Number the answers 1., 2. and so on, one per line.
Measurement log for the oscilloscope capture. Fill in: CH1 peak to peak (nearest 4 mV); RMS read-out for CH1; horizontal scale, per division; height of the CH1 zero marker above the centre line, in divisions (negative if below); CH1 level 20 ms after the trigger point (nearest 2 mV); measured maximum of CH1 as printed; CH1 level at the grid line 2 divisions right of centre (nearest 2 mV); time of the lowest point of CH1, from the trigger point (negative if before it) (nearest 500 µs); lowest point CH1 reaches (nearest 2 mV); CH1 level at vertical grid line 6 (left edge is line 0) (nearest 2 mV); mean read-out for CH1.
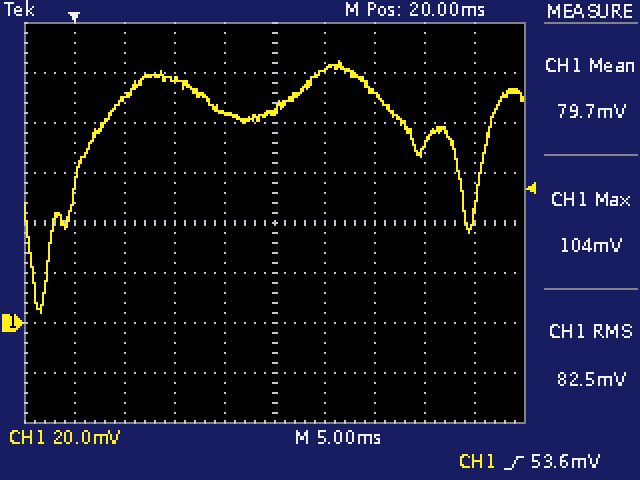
1. 100 mV
2. 82.5 mV
3. 5 ms
4. -2.0 div
5. 86 mV
6. 104 mV
7. 92 mV
8. -3.5 ms
9. 4 mV
10. 102 mV
11. 79.7 mV
